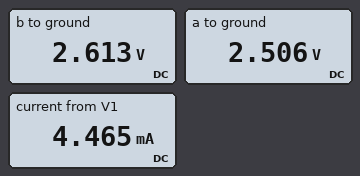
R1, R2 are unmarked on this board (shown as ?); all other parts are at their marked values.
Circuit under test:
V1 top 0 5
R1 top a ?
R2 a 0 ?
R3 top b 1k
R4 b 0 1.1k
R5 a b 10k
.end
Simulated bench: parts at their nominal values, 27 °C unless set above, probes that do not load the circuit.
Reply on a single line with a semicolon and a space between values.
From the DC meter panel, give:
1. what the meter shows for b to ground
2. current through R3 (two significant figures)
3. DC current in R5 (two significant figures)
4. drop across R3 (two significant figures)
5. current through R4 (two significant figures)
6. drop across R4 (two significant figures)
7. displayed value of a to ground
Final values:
2.613 V; 2.4 mA; 11 µA; 2.4 V; 2.4 mA; 2.6 V; 2.506 V
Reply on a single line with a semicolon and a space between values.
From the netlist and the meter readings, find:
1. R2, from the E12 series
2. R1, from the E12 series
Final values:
1.2 kΩ; 1.2 kΩ
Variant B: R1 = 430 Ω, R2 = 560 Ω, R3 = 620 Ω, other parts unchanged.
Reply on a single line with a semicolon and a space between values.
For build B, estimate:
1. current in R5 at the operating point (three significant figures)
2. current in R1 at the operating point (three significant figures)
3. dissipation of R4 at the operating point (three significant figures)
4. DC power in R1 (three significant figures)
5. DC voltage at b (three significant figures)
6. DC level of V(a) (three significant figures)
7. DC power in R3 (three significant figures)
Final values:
34.7 µA; 5.03 mA; 9.22 mW; 10.9 mW; 3.18 V; 2.84 V; 5.32 mW
